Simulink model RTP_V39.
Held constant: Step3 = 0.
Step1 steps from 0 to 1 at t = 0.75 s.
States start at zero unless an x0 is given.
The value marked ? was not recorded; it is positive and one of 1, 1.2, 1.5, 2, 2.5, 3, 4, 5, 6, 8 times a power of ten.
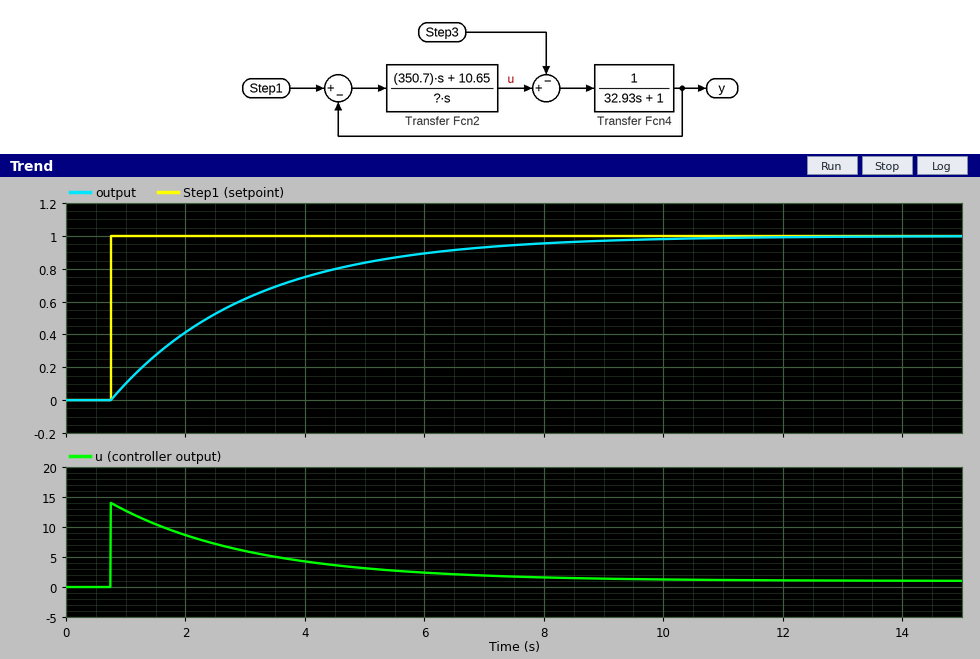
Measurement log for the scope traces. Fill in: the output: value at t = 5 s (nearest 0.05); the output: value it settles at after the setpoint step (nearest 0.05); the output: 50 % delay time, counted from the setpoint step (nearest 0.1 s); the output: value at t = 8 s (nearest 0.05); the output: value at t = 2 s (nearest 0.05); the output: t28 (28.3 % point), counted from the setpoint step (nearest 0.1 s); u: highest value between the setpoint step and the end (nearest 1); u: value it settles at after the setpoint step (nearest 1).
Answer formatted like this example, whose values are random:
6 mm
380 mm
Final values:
0.85
1.00
1.6 s
0.95
0.40
0.8 s
14
1
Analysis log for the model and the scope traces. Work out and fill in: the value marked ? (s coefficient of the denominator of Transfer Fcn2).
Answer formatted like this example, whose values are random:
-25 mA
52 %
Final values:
25
